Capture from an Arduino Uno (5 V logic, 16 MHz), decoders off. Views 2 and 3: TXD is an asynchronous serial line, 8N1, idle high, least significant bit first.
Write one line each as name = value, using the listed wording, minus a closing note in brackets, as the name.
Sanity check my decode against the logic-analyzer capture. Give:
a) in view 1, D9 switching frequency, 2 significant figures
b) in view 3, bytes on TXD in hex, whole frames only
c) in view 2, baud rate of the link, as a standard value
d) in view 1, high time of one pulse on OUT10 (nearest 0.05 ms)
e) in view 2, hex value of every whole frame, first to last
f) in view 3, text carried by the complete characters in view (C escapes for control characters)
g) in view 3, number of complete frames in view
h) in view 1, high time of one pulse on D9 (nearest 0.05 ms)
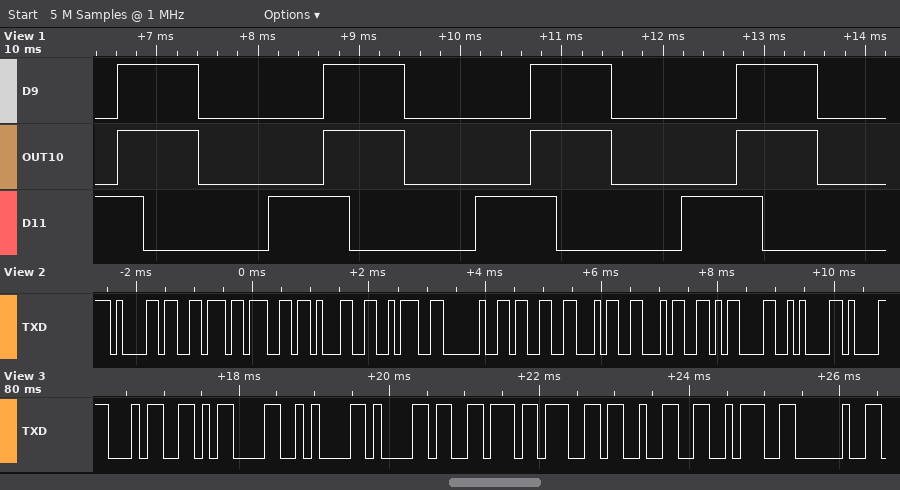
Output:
in view 1, D9 switching frequency, 2 significant figures = 490 Hz
in view 3, bytes on TXD in hex, whole frames only = 34 0D 0A 61 76 67 32 3A 20
in view 2, baud rate of the link, as a standard value = 9600 baud
in view 1, high time of one pulse on OUT10 = 0.80 ms
in view 2, hex value of every whole frame, first to last = 0x61 0x76 0x67 0x31 0x3A 0x20 0x33 0x34 0x34 0x0D 0x0A
in view 3, text carried by the complete characters in view = "4\r\navg2: "
in view 3, number of complete frames in view = 9
in view 1, high time of one pulse on D9 = 0.80 ms
